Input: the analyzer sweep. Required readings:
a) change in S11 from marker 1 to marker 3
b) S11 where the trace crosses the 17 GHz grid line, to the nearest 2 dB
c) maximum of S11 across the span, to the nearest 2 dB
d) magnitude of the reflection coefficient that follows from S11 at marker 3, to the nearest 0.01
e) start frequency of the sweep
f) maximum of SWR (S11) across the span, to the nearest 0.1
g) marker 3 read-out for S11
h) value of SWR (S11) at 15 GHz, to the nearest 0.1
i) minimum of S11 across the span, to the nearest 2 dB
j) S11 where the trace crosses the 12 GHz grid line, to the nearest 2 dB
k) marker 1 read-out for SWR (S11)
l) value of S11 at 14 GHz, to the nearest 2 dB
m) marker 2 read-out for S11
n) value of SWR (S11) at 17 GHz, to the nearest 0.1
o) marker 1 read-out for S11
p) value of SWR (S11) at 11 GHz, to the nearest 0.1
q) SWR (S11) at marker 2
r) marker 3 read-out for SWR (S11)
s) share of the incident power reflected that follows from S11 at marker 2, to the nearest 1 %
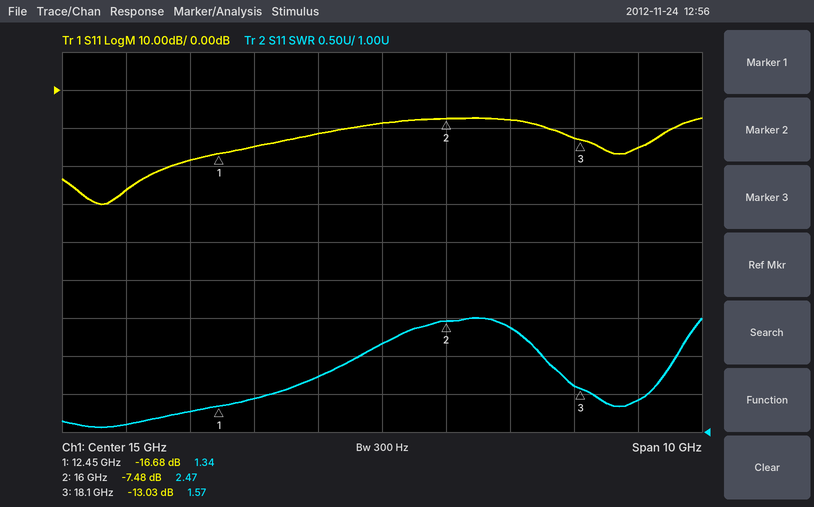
3.65 dB
-8 dB
-8 dB
0.22
10 GHz
2.5
-13.03 dB
2.2
-30 dB
-18 dB
1.34
-12 dB
-7.48 dB
2.4
-16.68 dB
1.1
2.47
1.57
18 %
